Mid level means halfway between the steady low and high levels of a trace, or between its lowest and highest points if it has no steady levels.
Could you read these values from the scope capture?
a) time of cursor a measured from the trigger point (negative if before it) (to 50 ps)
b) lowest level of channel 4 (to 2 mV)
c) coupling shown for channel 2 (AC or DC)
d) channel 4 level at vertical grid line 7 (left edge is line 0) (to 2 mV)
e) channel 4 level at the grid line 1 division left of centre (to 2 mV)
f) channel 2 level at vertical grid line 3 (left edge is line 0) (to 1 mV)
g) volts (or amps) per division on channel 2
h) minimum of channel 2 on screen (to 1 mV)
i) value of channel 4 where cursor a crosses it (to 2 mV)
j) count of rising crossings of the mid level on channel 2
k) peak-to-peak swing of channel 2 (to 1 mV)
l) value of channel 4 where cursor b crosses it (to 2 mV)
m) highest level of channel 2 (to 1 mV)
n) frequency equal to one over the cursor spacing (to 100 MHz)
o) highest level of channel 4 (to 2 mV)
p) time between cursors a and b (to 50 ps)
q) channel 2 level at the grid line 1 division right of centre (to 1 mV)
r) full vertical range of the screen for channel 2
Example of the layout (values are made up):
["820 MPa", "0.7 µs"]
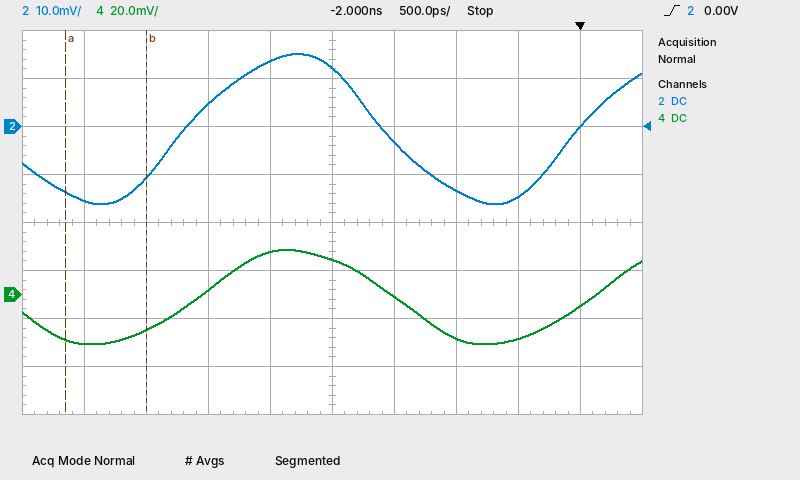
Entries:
["-4.15 ns", "-20 mV", "DC", "-18 mV", "18 mV", "5 mV", "10 mV", "-16 mV", "-18 mV", "2", "31 mV", "-14 mV", "15 mV", "1.5 GHz", "18 mV", "650 ps", "-3 mV", "80 mV"]
